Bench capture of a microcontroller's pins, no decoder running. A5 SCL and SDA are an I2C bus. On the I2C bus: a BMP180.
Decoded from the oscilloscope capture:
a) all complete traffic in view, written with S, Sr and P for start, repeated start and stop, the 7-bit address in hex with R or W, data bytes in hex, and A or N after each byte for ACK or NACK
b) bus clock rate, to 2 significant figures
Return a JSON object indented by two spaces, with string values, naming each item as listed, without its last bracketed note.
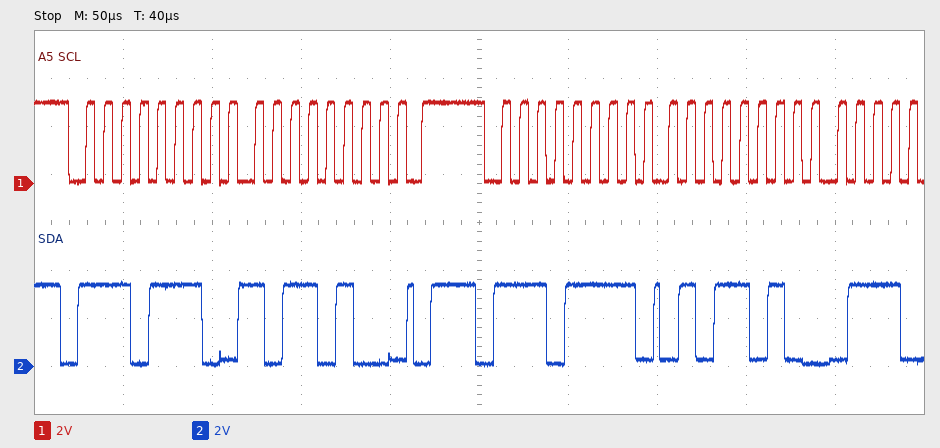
{
  "all complete traffic in view, written with S, Sr and P for start, repeated start and stop, the 7-bit address in hex with R or W, data bytes in hex, and A or N after each byte for ACK or NACK": "S 77W A B4 A P S 77R A 5A A",
  "bus clock rate, to 2 significant figures": "100 kHz"
}
